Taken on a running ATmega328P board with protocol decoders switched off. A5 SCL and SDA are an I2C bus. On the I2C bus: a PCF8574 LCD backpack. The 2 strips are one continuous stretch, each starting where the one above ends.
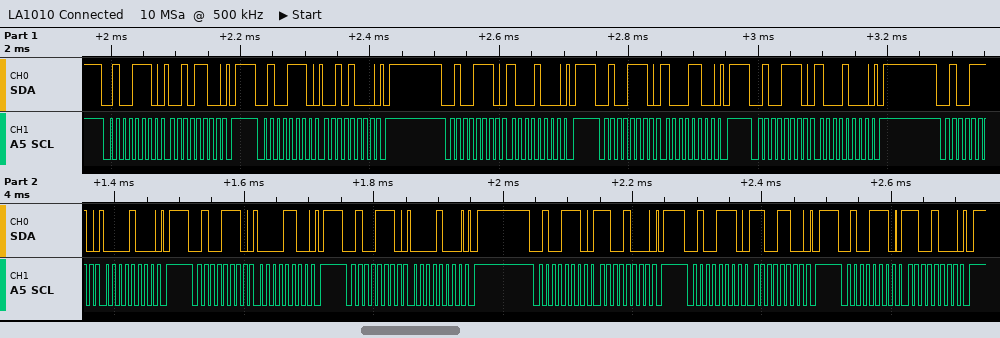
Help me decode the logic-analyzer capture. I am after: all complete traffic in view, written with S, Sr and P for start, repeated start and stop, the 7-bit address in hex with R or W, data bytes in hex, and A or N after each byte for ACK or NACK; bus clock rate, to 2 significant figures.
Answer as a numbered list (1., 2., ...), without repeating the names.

1. S 27W A 2C A P S 27W A 28 A P S 27W A 88 A P S 27W A 8C A P S 27W A 88 A P S 27W A 08 A P S 27W A 0C A P S 27W A 08 A P S 27W A C8 A P S 27W A CC A P S 27W A C8 A P
2. 100 kHz
